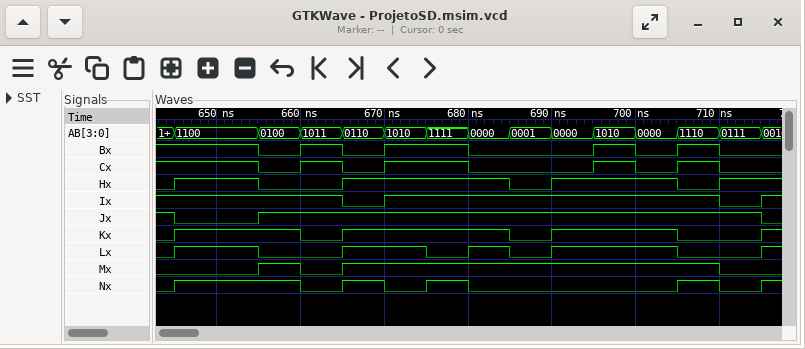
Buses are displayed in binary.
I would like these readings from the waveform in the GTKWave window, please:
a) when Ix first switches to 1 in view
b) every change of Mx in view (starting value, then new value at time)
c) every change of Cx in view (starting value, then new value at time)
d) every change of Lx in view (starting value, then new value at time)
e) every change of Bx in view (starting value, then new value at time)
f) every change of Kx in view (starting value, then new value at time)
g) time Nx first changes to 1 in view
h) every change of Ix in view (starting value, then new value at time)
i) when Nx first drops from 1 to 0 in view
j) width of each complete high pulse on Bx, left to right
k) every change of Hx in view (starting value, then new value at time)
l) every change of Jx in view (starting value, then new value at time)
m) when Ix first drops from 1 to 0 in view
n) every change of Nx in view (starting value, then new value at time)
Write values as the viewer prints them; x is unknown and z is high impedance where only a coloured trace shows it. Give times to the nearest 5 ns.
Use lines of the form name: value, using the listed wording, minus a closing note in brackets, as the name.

when Ix first switches to 1 in view: 670 ns
every change of Mx in view: 0, 1 at 655 ns, 0 at 660 ns, 1 at 665 ns, 0 at 710 ns
every change of Cx in view: 1, 0 at 655 ns, 1 at 660 ns, 0 at 665 ns, 1 at 670 ns, 0 at 680 ns, 1 at 695 ns, 0 at 700 ns, 1 at 705 ns, 0 at 710 ns
every change of Lx in view: 0, 1 at 645 ns, 0 at 655 ns, 1 at 665 ns, 0 at 675 ns, 1 at 680 ns, 0 at 685 ns, 1 at 690 ns, 0 at 705 ns, 1 at 715 ns
every change of Bx in view: 1, 0 at 655 ns, 1 at 660 ns, 0 at 665 ns, 1 at 670 ns, 0 at 680 ns, 1 at 695 ns, 0 at 700 ns, 1 at 705 ns, 0 at 710 ns
every change of Kx in view: 0, 1 at 645 ns, 0 at 660 ns, 1 at 665 ns, 0 at 685 ns, 1 at 690 ns, 0 at 705 ns, 1 at 715 ns
time Nx first changes to 1 in view: 645 ns
every change of Ix in view: 1, 0 at 665 ns, 1 at 670 ns, 0 at 710 ns, 1 at 715 ns
when Nx first drops from 1 to 0 in view: 660 ns
width of each complete high pulse on Bx, left to right: 5 ns, 10 ns, 5 ns, 5 ns
every change of Hx in view: 0, 1 at 645 ns, 0 at 655 ns, 1 at 665 ns, 0 at 685 ns, 1 at 690 ns, 0 at 705 ns, 1 at 710 ns
every change of Jx in view: 1, 0 at 645 ns, 1 at 655 ns, 0 at 715 ns
when Ix first drops from 1 to 0 in view: 665 ns
every change of Nx in view: 0, 1 at 645 ns, 0 at 660 ns, 1 at 665 ns, 0 at 670 ns, 1 at 675 ns, 0 at 680 ns, 1 at 705 ns, 0 at 710 ns, 1 at 715 ns
